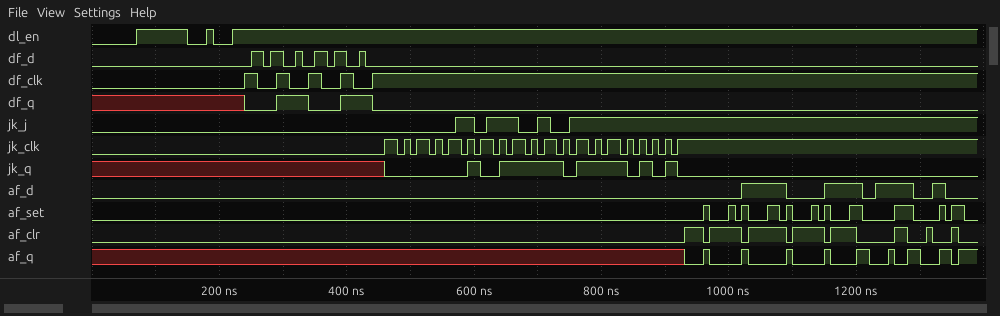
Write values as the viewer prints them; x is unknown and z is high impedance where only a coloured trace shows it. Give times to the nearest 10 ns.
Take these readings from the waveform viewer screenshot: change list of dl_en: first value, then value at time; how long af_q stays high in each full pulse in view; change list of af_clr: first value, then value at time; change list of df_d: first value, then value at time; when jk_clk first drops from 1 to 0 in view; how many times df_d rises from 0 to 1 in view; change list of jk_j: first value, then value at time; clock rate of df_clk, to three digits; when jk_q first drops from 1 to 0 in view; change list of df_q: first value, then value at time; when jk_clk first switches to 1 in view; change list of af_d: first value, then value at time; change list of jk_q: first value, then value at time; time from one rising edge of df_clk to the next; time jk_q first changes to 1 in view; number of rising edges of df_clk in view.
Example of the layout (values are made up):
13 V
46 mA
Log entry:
0, 1 at 70 ns, 0 at 150 ns, 1 at 180 ns, 0 at 190 ns, 1 at 220 ns
10 ns, 10 ns, 10 ns, 10 ns, 20 ns, 10 ns, 20 ns, 20 ns
0, 1 at 930 ns, 0 at 960 ns, 1 at 970 ns, 0 at 1020 ns, 1 at 1030 ns, 0 at 1090 ns, 1 at 1100 ns, 0 at 1150 ns, 1 at 1160 ns, 0 at 1200 ns, 1 at 1260 ns, 0 at 1280 ns, 1 at 1310 ns, 0 at 1320 ns, 1 at 1350 ns, 0 at 1360 ns
0, 1 at 250 ns, 0 at 270 ns, 1 at 280 ns, 0 at 300 ns, 1 at 320 ns, 0 at 330 ns, 1 at 350 ns, 0 at 370 ns, 1 at 380 ns, 0 at 400 ns, 1 at 420 ns, 0 at 430 ns
480 ns
6
0, 1 at 570 ns, 0 at 600 ns, 1 at 620 ns, 0 at 670 ns, 1 at 700 ns, 0 at 720 ns, 1 at 750 ns
20.0 MHz
610 ns
x, 0 at 240 ns, 1 at 290 ns, 0 at 340 ns, 1 at 390 ns, 0 at 440 ns
460 ns
0, 1 at 1020 ns, 0 at 1090 ns, 1 at 1150 ns, 0 at 1210 ns, 1 at 1230 ns, 0 at 1290 ns, 1 at 1320 ns, 0 at 1340 ns
x, 0 at 460 ns, 1 at 590 ns, 0 at 610 ns, 1 at 640 ns, 0 at 740 ns, 1 at 760 ns, 0 at 840 ns, 1 at 860 ns, 0 at 880 ns, 1 at 900 ns, 0 at 920 ns
50 ns
590 ns
5
